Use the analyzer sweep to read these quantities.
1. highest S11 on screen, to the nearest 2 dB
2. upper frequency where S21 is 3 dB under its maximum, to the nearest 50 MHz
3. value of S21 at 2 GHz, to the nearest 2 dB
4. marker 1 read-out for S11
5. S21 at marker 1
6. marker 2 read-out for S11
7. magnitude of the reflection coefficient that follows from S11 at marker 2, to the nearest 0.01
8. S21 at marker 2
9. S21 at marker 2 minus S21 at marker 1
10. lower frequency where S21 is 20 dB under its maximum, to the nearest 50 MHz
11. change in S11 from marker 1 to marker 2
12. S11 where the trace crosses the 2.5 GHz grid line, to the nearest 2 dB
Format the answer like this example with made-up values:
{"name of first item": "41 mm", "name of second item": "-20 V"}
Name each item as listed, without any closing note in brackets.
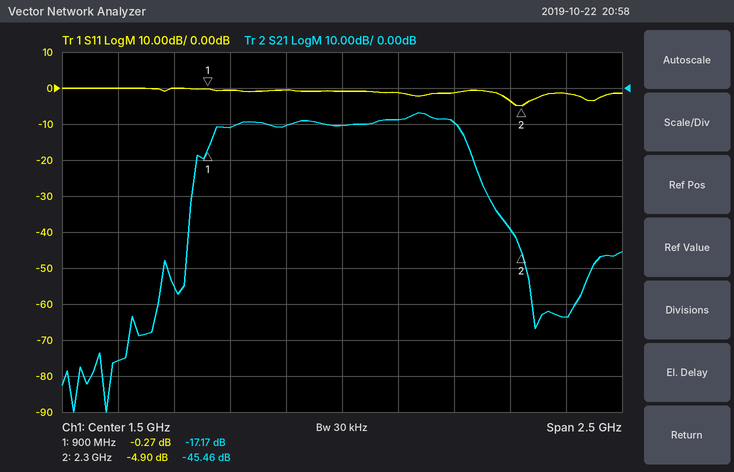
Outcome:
{"highest S11 on screen, to the nearest 2 dB": "0 dB", "upper frequency where S21 is 3 dB under its maximum, to the nearest 50 MHz": "2.00 GHz", "value of S21 at 2 GHz, to the nearest 2 dB": "-10 dB", "marker 1 read-out for S11": "-0.27 dB", "S21 at marker 1": "-17.17 dB", "marker 2 read-out for S11": "-4.90 dB", "magnitude of the reflection coefficient that follows from S11 at marker 2, to the nearest 0.01": "0.57", "S21 at marker 2": "-45.46 dB", "S21 at marker 2 minus S21 at marker 1": "-28.29 dB", "lower frequency where S21 is 20 dB under its maximum, to the nearest 50 MHz": "850 MHz", "change in S11 from marker 1 to marker 2": "-4.63 dB", "S11 where the trace crosses the 2.5 GHz grid line, to the nearest 2 dB": "-2 dB"}
